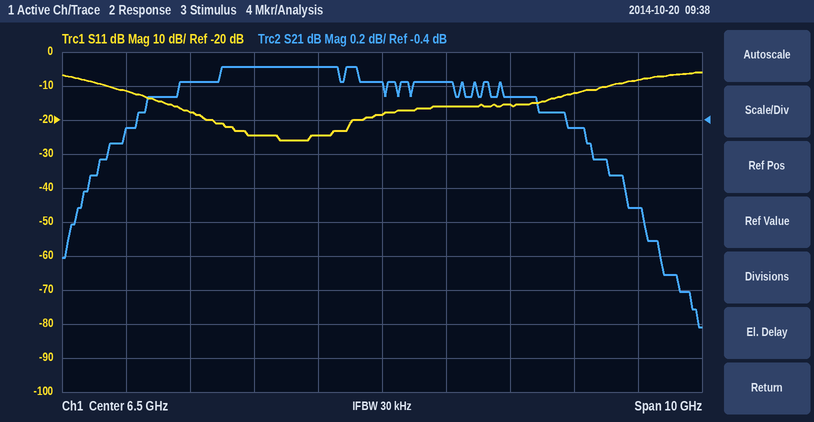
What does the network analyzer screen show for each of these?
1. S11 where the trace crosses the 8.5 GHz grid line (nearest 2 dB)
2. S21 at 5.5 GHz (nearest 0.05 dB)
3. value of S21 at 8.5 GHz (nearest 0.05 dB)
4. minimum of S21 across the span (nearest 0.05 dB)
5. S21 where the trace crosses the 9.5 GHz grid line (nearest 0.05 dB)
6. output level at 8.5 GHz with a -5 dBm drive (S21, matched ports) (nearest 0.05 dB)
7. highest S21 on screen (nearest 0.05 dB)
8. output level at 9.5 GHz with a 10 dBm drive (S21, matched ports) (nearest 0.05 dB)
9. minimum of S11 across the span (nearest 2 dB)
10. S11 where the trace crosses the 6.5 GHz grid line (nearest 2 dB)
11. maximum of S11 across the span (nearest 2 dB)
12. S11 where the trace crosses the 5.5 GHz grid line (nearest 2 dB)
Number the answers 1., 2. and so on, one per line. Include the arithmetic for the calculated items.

1. -16 dB
2. -0.10 dB
3. -0.25 dB
4. -1.60 dB
5. -0.45 dB
6. -5 dBm + (-0.25 dB) = -5.25 dBm
7. -0.10 dB
8. 10 dBm + (-0.45 dB) = 9.55 dBm
9. -26 dB
10. -18 dB
11. -6 dB
12. -24 dB
